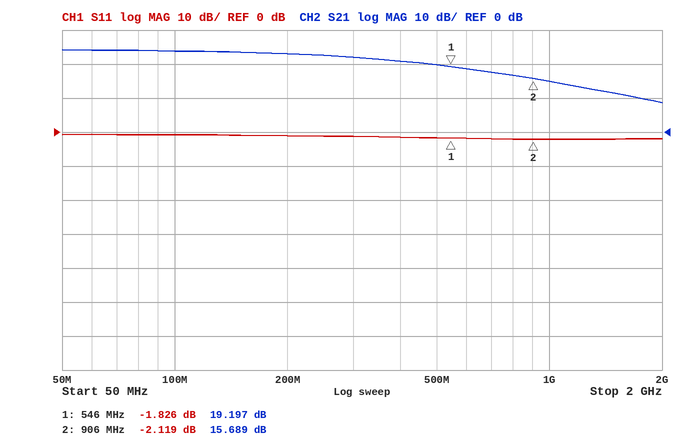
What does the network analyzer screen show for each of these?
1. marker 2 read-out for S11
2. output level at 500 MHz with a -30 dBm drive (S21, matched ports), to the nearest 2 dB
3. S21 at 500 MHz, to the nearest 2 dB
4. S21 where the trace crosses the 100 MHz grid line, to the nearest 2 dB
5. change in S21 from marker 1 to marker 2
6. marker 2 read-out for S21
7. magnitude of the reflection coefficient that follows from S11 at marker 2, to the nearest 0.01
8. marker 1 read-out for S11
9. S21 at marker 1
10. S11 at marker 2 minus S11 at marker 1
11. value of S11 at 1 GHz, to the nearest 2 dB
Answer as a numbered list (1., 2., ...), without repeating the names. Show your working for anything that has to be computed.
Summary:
1. -2.119 dB
2. -30 dBm + (20 dB) = -10 dBm
3. 20 dB
4. 24 dB
5. 15.689 − (19.197) = -3.508 dB
6. 15.689 dB
7. 10^(-2.119/20) ≈ 0.78
8. -1.826 dB
9. 19.197 dB
10. -2.119 − (-1.826) = -0.293 dB
11. -2 dB
